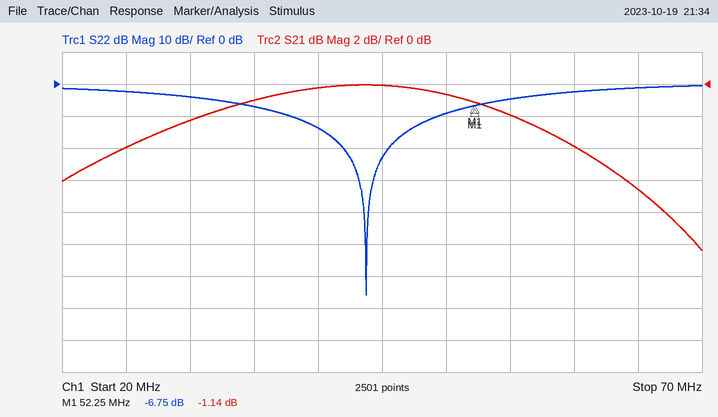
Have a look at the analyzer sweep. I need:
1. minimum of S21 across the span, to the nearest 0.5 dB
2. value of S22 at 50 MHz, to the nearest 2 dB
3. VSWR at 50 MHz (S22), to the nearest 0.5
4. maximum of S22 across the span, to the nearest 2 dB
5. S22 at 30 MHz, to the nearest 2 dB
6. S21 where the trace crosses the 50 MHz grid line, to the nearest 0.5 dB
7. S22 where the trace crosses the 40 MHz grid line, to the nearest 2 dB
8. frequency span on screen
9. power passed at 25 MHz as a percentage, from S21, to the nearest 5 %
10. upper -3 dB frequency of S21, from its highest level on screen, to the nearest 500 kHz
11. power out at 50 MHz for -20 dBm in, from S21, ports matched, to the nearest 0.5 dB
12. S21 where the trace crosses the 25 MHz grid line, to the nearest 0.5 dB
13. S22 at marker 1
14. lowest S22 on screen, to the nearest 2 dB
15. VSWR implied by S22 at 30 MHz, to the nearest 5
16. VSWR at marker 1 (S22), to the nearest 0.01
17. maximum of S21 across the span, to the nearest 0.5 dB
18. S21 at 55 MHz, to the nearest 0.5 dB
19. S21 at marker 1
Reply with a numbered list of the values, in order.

1. -10.5 dB
2. -10 dB
3. 2.0
4. 0 dB
5. -4 dB
6. -0.5 dB
7. -14 dB
8. 50 MHz
9. 40 %
10. 58.0 MHz
11. -20.5 dBm
12. -4.0 dB
13. -6.75 dB
14. -66 dB
15. 5
16. 2.70
17. 0.0 dB
18. -2.0 dB
19. -1.14 dB
